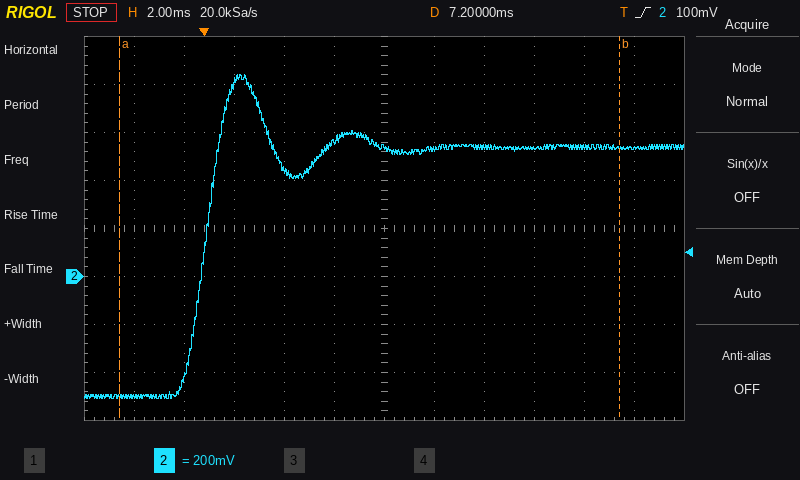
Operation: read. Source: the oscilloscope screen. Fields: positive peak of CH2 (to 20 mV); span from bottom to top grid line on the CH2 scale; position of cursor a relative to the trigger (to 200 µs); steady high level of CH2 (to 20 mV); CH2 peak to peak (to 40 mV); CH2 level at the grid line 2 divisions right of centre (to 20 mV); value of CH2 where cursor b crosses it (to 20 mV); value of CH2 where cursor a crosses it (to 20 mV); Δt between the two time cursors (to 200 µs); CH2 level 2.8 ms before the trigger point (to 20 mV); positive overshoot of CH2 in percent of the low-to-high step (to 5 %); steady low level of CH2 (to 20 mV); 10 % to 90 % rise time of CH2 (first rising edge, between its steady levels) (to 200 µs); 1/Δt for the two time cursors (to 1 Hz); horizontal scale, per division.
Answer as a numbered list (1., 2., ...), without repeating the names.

1. 840 mV
2. 1.6 V
3. -3.4 ms
4. 540 mV
5. 1.36 V
6. 540 mV
7. 540 mV
8. -500 mV
9. 20.0 ms
10. -500 mV
11. 30 %
12. -500 mV
13. 1.2 ms
14. 50 Hz
15. 2 ms
